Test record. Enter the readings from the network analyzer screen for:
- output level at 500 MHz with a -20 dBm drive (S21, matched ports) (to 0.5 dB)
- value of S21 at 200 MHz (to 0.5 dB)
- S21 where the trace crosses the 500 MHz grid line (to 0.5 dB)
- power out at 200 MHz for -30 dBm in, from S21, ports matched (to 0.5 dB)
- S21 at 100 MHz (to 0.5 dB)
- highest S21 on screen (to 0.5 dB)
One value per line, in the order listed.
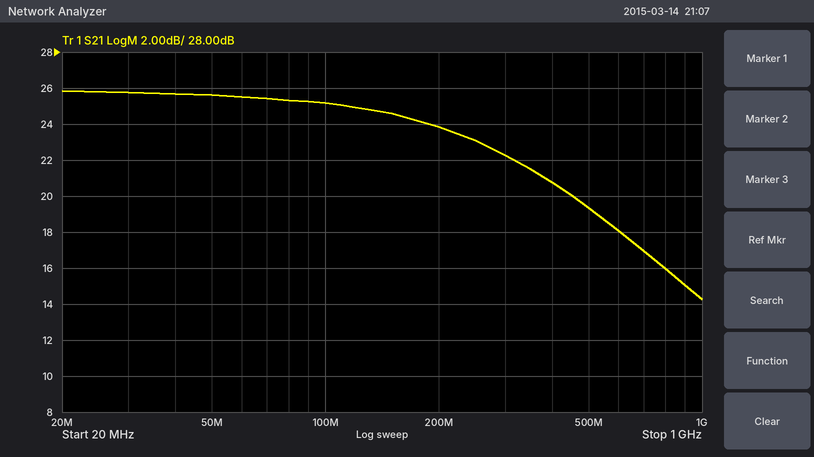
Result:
-0.5 dBm
24.0 dB
19.5 dB
-6.0 dBm
25.0 dB
26.0 dB
